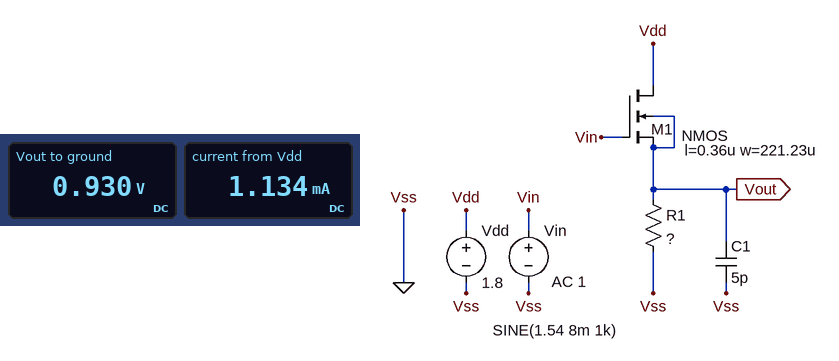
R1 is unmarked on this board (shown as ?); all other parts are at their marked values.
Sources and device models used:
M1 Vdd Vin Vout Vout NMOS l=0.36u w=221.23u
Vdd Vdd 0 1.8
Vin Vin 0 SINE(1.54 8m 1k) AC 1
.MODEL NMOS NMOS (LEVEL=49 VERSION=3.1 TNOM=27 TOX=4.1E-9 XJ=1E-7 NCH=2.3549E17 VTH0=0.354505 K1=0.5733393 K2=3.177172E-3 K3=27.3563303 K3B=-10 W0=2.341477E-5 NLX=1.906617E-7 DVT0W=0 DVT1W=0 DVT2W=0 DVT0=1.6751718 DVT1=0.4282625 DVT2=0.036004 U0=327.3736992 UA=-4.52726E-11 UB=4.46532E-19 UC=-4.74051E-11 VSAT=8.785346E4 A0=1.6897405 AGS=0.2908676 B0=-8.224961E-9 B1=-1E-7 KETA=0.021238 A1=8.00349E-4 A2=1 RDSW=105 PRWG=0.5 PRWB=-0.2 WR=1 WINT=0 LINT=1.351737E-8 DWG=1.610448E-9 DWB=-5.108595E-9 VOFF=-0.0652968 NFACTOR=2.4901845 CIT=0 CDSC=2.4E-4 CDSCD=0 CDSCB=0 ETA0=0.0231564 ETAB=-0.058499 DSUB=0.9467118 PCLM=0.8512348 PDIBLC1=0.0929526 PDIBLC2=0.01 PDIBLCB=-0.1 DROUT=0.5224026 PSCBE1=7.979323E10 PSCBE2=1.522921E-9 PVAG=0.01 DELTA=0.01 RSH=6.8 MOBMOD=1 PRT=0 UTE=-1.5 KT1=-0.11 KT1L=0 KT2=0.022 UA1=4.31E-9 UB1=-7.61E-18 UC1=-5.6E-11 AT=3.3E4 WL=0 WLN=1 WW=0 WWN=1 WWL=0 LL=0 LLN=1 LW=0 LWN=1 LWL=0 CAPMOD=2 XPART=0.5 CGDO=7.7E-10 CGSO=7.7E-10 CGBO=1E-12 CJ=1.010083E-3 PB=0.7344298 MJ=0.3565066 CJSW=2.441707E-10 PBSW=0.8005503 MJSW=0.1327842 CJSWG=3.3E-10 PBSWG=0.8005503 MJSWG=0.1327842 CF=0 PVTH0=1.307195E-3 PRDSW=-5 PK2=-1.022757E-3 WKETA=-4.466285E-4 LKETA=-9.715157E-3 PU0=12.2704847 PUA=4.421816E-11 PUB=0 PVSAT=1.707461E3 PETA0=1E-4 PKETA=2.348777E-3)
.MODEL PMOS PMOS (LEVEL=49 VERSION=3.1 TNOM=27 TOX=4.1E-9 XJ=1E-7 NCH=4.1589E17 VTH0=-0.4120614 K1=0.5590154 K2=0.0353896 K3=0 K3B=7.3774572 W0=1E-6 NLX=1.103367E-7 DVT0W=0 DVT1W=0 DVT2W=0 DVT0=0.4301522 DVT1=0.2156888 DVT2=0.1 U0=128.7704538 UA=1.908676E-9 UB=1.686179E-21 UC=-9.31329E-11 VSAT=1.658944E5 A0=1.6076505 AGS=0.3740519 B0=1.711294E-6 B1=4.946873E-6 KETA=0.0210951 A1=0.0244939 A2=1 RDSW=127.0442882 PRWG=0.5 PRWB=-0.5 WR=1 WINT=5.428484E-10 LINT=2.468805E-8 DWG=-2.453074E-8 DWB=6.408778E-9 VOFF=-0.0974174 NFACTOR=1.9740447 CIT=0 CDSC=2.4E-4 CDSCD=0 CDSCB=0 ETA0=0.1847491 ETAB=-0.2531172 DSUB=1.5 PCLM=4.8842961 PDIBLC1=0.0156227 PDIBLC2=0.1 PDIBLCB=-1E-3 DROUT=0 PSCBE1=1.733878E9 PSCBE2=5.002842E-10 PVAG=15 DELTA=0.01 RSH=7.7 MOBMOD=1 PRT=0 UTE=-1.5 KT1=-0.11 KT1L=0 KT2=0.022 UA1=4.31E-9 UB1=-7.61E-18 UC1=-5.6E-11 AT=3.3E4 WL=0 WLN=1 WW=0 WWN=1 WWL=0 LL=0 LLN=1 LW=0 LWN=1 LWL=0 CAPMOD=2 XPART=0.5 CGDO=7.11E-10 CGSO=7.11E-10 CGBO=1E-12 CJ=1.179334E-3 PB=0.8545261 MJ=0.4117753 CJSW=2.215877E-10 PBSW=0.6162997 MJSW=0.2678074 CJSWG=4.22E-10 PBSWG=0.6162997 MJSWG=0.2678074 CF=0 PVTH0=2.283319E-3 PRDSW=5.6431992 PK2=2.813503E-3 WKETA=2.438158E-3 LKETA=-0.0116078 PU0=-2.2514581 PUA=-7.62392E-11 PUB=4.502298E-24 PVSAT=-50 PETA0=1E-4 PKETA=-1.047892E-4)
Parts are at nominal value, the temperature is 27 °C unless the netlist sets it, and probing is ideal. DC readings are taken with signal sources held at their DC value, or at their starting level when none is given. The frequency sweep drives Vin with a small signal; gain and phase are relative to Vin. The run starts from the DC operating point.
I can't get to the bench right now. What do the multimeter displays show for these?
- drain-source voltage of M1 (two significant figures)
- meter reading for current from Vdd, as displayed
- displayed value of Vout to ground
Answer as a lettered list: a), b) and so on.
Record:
a) 870 mV
b) 1.134 mA
c) 0.930 V
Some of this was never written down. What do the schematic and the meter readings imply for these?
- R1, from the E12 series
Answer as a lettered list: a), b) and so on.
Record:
a) 820 Ω
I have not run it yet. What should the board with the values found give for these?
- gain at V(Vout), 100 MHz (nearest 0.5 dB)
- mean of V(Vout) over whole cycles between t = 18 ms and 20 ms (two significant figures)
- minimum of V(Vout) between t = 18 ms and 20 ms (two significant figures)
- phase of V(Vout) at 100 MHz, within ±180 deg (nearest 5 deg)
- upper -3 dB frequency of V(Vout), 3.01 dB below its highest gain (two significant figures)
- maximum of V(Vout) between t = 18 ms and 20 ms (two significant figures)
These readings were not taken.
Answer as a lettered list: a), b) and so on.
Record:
a) -1.0 dB
b) 930 mV
c) 920 mV
d) -10 deg
e) 490 MHz
f) 940 mV
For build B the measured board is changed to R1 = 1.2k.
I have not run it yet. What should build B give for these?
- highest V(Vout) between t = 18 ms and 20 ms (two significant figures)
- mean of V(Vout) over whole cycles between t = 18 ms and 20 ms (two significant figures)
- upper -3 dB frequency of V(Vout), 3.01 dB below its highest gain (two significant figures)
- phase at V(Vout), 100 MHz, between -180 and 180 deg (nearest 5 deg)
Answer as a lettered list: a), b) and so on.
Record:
a) 960 mV
b) 950 mV
c) 390 MHz
d) -15 deg
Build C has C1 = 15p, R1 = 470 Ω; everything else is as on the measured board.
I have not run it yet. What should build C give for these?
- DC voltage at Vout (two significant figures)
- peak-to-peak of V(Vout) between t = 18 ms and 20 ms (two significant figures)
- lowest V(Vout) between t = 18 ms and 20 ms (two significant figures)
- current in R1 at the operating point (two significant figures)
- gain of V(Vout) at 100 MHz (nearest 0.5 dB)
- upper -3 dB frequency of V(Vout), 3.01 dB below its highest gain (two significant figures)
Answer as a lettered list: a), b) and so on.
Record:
a) 890 mV
b) 14 mV
c) 880 mV
d) 1.9 mA
e) -1.5 dB
f) 230 MHz
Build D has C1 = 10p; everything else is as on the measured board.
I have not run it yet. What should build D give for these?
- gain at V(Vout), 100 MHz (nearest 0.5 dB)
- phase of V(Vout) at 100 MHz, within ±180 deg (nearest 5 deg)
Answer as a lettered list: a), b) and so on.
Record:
a) -1.5 dB
b) -20 deg
